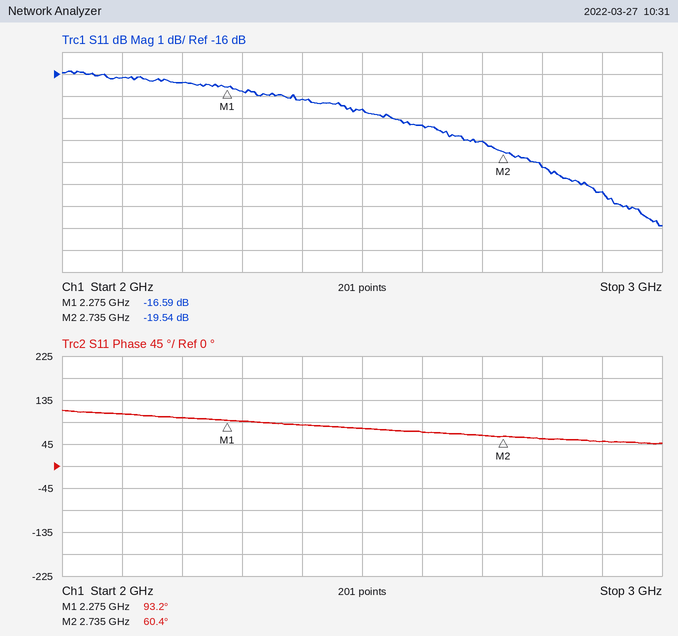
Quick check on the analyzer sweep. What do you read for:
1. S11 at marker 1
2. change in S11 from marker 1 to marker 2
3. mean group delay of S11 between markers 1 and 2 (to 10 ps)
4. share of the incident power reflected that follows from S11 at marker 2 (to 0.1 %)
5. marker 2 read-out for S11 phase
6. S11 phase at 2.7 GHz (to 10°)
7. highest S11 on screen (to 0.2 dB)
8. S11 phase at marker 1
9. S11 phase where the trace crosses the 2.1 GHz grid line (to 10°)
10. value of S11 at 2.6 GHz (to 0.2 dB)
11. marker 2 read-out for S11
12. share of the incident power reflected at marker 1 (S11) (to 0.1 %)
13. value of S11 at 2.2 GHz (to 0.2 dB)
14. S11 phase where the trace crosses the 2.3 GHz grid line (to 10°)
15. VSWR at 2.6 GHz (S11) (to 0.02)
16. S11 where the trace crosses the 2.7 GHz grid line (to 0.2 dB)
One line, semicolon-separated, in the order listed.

-16.59 dB; -2.95 dB; 200 ps; 1.1 %; 60.4°; 60°; -15.8 dB; 93.2°; 110°; -18.4 dB; -19.54 dB; 2.2 %; -16.4 dB; 90°; 1.28; -19.0 dB
